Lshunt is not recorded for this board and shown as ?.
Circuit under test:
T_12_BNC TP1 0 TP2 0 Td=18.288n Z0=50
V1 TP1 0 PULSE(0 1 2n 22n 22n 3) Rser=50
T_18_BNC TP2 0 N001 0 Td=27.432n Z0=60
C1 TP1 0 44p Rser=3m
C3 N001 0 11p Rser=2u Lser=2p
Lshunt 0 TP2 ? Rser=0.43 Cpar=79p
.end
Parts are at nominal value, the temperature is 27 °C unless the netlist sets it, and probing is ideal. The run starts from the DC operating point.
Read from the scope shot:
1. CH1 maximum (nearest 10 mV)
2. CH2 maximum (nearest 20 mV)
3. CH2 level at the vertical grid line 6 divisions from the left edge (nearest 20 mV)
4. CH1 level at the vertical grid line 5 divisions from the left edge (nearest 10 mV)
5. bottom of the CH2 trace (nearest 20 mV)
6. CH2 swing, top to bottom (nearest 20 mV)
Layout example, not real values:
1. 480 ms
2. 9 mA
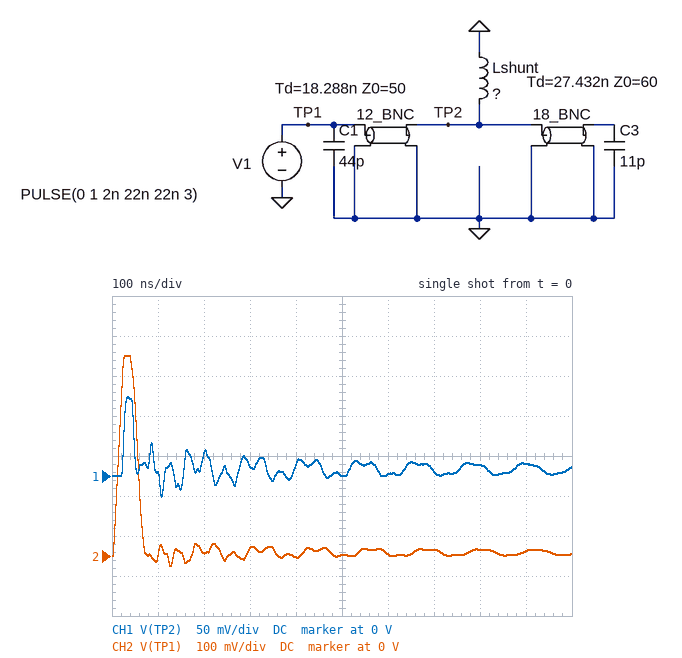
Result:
1. 100 mV
2. 500 mV
3. 0 V
4. 0 V
5. -20 mV
6. 520 mV
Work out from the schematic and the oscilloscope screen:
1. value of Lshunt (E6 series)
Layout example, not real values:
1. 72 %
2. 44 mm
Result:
1. 100 nH
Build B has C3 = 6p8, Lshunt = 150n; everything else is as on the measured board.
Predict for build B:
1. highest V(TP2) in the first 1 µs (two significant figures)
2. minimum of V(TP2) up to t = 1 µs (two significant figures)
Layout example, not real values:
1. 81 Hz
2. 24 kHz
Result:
1. 140 mV
2. -46 mV
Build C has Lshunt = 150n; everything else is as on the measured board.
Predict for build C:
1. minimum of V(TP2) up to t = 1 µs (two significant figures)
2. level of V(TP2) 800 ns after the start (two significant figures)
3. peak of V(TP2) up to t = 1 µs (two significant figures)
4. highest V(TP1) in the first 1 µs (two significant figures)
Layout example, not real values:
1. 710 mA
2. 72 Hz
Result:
1. -46 mV
2. 21 mV
3. 140 mV
4. 500 mV
